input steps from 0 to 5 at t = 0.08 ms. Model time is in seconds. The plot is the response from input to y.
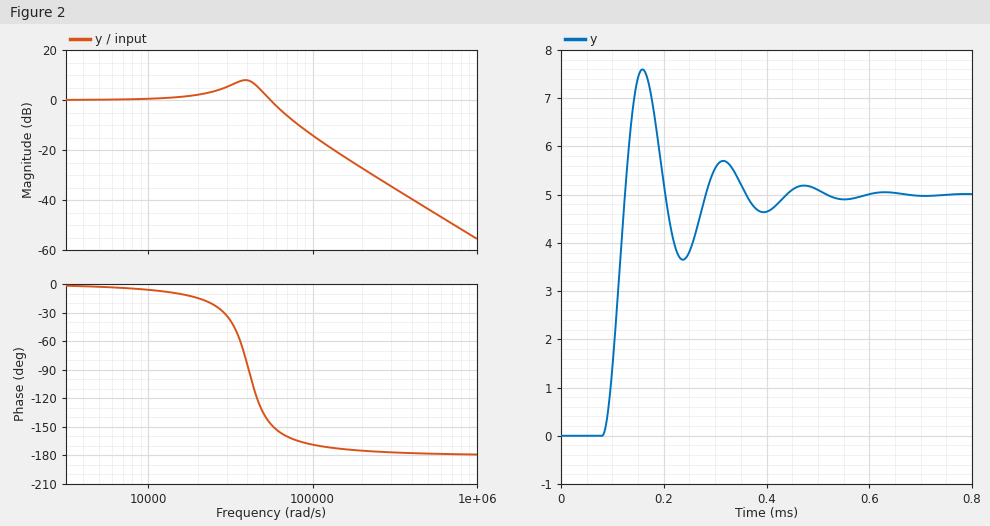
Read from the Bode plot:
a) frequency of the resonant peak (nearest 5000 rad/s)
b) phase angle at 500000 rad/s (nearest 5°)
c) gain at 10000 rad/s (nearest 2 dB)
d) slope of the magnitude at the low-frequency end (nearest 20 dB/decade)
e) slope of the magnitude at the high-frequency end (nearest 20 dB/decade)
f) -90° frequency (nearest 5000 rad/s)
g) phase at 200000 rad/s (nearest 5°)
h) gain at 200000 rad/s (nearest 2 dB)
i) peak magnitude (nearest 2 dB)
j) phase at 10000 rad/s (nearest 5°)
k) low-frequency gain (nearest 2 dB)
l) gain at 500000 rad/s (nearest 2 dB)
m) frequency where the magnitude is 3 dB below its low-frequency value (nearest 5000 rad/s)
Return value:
40000 rad/s
-180°
0 dB
0 dB/decade
-40 dB/decade
40000 rad/s
-175°
-28 dB
8 dB
-5°
0 dB
-44 dB
60000 rad/s
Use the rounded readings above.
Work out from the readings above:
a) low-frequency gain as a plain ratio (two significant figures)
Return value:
1.0
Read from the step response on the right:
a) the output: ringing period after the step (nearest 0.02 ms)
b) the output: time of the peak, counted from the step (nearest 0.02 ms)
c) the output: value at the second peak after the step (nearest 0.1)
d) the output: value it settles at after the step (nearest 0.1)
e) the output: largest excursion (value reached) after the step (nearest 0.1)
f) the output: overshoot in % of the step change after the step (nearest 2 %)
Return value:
0.16 ms
0.08 ms
5.7
5.0
7.6
52 %
